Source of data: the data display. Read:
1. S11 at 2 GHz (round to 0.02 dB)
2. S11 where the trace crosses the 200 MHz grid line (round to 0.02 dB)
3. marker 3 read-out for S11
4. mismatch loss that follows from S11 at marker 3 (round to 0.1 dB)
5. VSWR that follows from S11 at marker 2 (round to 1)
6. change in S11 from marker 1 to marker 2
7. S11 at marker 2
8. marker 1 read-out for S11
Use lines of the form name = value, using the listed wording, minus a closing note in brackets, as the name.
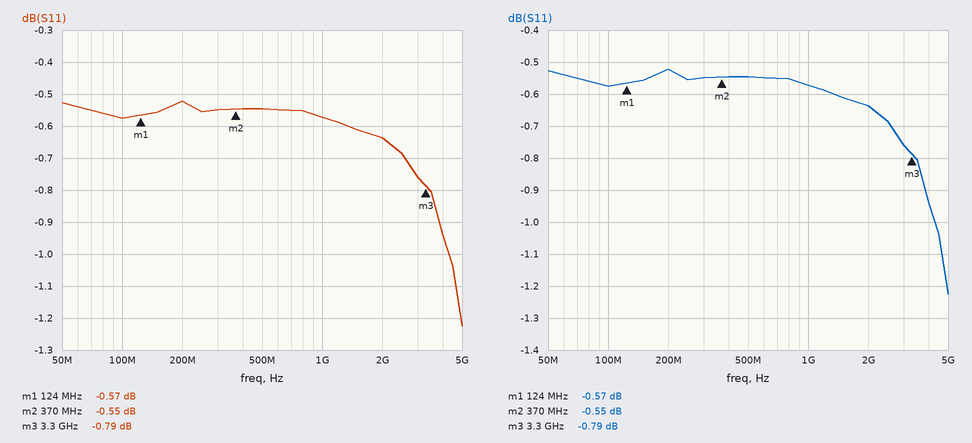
S11 at 2 GHz = -0.64 dB
S11 where the trace crosses the 200 MHz grid line = -0.52 dB
marker 3 read-out for S11 = -0.79 dB
mismatch loss that follows from S11 at marker 3 = 7.8 dB
VSWR that follows from S11 at marker 2 = 32
change in S11 from marker 1 to marker 2 = 0.02 dB
S11 at marker 2 = -0.55 dB
marker 1 read-out for S11 = -0.57 dB
